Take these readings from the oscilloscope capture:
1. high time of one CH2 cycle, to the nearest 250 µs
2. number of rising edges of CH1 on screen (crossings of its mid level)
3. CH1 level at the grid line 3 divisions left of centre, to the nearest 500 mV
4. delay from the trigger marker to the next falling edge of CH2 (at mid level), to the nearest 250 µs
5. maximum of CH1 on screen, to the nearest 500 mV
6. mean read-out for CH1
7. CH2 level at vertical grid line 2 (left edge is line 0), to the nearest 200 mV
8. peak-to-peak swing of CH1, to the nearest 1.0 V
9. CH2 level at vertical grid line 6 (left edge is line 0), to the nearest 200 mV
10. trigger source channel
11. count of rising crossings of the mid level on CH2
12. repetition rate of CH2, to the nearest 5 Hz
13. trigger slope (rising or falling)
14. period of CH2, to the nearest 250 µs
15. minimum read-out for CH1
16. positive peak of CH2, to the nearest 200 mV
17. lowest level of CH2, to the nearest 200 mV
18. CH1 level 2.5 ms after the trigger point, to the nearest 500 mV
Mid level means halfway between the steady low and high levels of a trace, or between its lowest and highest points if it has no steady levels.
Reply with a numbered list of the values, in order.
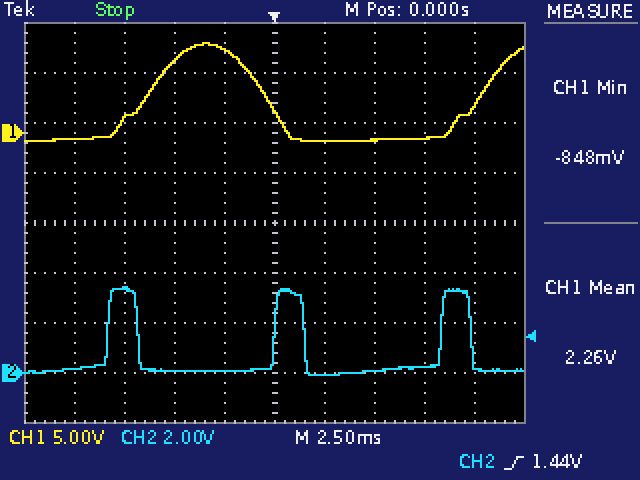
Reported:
1. 1.50 ms
2. 2
3. 1.5 V
4. 1.50 ms
5. 9.0 V
6. 2.26 V
7. 3.4 V
8. 10.0 V
9. 0.0 V
10. CH2
11. 3
12. 120 Hz
13. rising
14. 8.25 ms
15. -848 mV
16. 3.4 V
17. 0.0 V
18. -1.0 V
